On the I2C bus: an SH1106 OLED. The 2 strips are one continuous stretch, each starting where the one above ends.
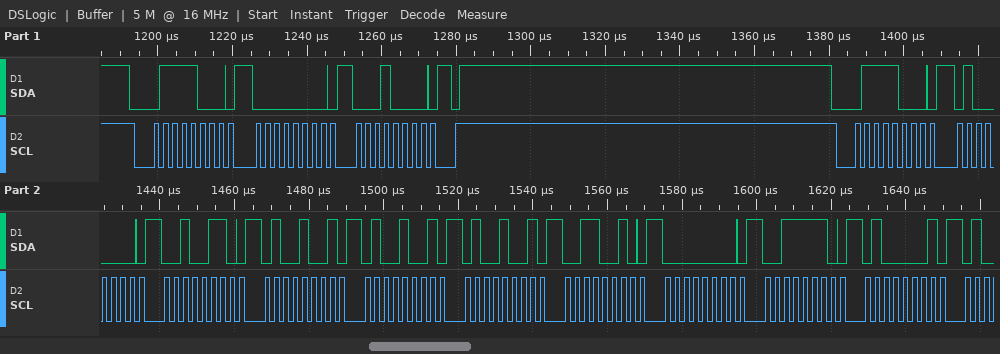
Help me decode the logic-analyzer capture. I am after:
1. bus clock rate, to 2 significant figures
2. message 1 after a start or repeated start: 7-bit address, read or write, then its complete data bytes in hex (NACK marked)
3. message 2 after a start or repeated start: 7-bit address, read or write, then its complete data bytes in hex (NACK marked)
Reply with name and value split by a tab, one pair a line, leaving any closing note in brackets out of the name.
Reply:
bus clock rate, to 2 significant figures	400 kHz
message 1 after a start or repeated start: 7-bit address, read or write, then its complete data bytes in hex	0x3C write: 00 10
message 2 after a start or repeated start: 7-bit address, read or write, then its complete data bytes in hex	0x3C write: 40 26 49 49 49 32 00 3E 41
